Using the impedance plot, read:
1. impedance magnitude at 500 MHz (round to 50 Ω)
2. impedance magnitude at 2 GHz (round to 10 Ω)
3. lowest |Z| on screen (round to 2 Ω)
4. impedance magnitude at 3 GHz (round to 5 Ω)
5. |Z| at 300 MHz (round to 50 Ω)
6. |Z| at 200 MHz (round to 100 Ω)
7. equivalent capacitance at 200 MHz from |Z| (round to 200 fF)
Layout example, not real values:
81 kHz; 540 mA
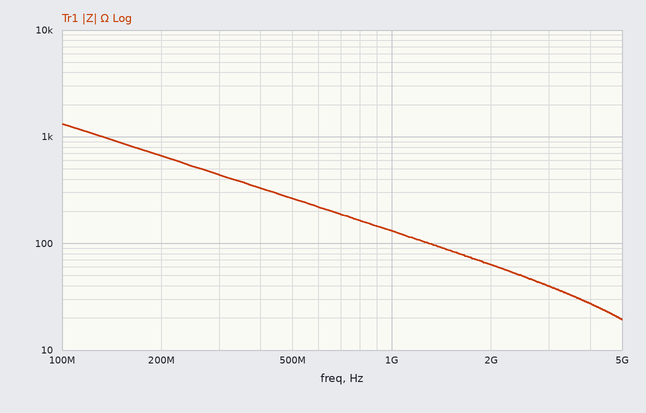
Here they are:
250 Ω; 60 Ω; 20 Ω; 40 Ω; 450 Ω; 700 Ω; 1.2 pF
